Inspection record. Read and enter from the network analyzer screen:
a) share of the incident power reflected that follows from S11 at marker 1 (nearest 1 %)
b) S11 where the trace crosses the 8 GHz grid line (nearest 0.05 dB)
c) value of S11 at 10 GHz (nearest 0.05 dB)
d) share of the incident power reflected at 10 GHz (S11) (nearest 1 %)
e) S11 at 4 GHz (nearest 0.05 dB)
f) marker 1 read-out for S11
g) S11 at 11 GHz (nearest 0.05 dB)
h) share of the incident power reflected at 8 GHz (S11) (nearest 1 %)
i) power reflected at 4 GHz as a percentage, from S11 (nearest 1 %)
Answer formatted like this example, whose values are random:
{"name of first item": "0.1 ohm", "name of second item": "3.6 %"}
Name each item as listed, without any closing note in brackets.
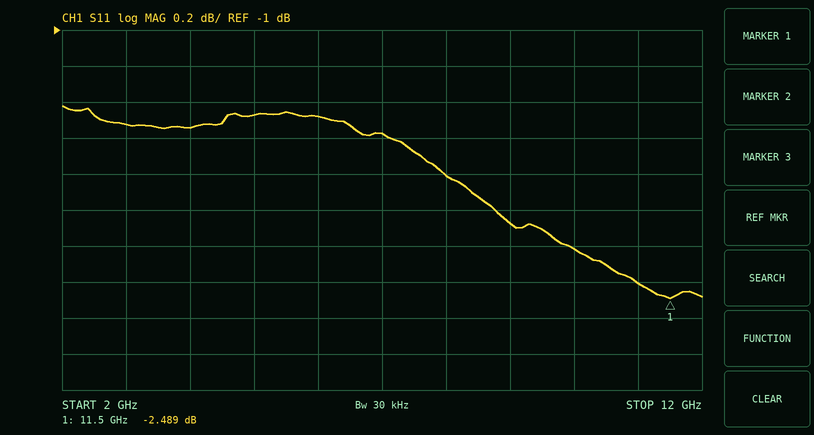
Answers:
{"share of the incident power reflected that follows from S11 at marker 1": "56 %", "S11 where the trace crosses the 8 GHz grid line": "-1.80 dB", "value of S11 at 10 GHz": "-2.20 dB", "share of the incident power reflected at 10 GHz (S11)": "60 %", "S11 at 4 GHz": "-1.55 dB", "marker 1 read-out for S11": "-2.489 dB", "S11 at 11 GHz": "-2.40 dB", "share of the incident power reflected at 8 GHz (S11)": "66 %", "power reflected at 4 GHz as a percentage, from S11": "70 %"}
